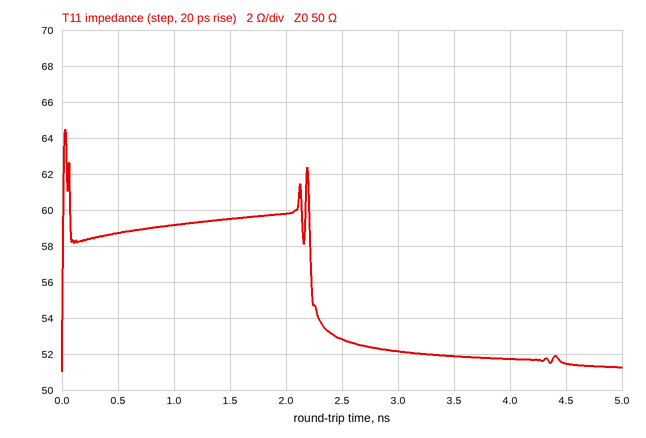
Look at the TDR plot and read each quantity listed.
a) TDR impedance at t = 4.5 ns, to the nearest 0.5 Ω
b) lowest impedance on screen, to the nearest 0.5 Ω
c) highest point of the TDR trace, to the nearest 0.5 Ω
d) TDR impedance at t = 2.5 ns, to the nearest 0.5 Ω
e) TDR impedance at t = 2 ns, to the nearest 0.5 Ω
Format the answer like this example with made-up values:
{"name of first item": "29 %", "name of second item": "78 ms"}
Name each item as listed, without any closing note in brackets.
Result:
{"TDR impedance at t = 4.5 ns, to the nearest 0.5 Ω": "51.5 Ω", "lowest impedance on screen, to the nearest 0.5 Ω": "51.0 Ω", "highest point of the TDR trace, to the nearest 0.5 Ω": "64.5 Ω", "TDR impedance at t = 2.5 ns, to the nearest 0.5 Ω": "53.0 Ω", "TDR impedance at t = 2 ns, to the nearest 0.5 Ω": "60.0 Ω"}
